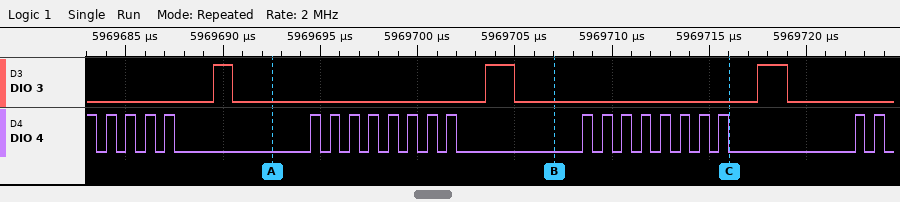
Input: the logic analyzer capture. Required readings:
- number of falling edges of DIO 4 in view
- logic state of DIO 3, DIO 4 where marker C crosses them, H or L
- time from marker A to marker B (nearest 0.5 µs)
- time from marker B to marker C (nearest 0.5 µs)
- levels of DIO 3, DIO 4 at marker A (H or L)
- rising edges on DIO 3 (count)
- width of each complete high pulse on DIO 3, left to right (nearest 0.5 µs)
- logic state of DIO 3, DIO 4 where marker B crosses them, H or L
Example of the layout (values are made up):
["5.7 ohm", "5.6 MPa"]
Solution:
["23", "DIO 3=L, DIO 4=L", "14.5 µs", "9 µs", "DIO 3=L, DIO 4=L", "3", "1 µs, 1.5 µs, 1.5 µs", "DIO 3=L, DIO 4=L"]
